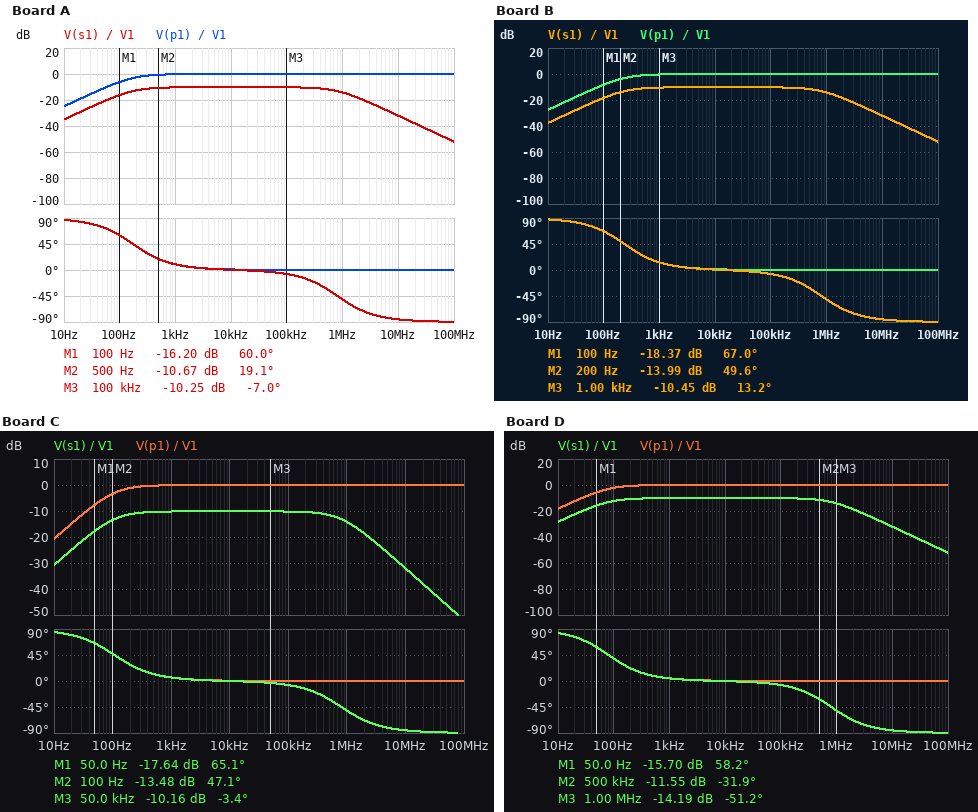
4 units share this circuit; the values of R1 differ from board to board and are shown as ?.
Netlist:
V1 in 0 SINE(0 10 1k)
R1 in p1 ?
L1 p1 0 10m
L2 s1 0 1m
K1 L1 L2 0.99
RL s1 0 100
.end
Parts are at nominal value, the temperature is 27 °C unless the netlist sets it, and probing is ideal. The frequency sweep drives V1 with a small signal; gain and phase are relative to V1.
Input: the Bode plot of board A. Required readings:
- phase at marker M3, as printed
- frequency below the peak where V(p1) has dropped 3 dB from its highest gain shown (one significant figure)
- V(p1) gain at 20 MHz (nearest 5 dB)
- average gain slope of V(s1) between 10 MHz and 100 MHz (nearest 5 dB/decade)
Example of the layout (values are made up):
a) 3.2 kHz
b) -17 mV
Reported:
a) -7.0 deg
b) 200 Hz
c) 0 dB
d) -20 dB/decade
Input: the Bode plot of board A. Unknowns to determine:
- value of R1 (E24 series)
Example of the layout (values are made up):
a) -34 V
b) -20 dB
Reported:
a) 11 Ω
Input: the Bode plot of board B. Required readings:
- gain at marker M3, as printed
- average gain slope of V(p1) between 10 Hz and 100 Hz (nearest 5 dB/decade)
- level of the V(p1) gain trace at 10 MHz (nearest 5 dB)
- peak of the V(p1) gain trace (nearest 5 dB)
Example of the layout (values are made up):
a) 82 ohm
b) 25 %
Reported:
a) -10.45 dB
b) 20 dB/decade
c) 0 dB
d) 0 dB
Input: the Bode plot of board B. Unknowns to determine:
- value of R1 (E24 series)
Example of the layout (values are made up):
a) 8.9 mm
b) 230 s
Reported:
a) 15 Ω
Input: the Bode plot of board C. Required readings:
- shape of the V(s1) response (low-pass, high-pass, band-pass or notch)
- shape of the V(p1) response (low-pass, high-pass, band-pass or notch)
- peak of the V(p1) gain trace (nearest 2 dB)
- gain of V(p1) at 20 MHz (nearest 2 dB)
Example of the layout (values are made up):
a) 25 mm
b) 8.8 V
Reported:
a) band-pass
b) high-pass
c) 0 dB
d) 0 dB
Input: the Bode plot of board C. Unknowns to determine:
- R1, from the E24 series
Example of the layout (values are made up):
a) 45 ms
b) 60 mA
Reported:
a) 6.8 Ω
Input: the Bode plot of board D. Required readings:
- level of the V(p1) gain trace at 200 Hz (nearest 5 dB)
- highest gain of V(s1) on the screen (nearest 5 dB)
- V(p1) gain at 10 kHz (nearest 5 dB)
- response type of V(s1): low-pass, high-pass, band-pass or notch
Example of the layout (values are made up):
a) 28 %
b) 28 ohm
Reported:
a) 0 dB
b) -10 dB
c) 0 dB
d) band-pass
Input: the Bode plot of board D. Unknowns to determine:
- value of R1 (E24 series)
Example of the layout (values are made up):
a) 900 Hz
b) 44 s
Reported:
a) 5.1 Ω
